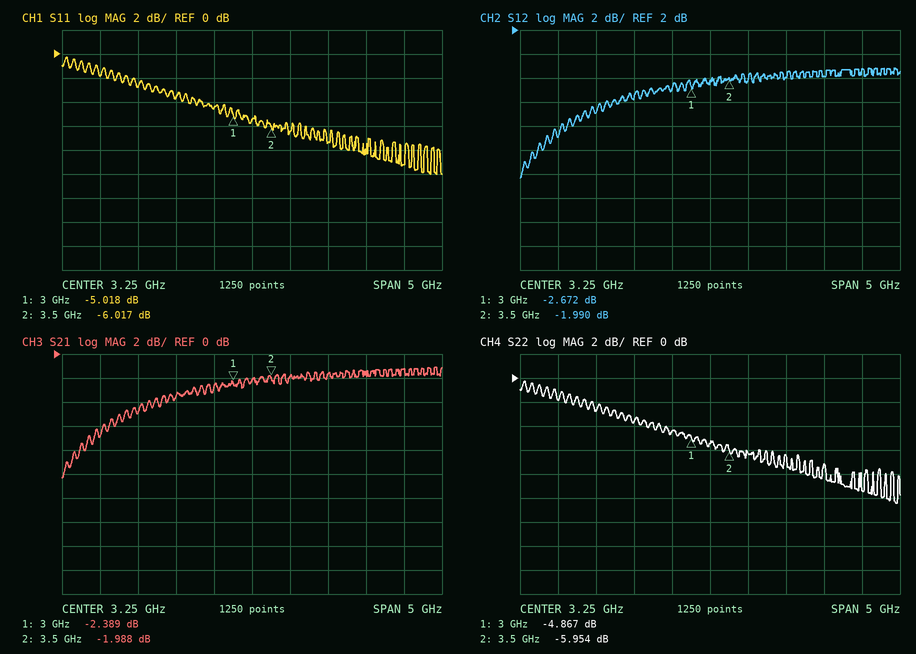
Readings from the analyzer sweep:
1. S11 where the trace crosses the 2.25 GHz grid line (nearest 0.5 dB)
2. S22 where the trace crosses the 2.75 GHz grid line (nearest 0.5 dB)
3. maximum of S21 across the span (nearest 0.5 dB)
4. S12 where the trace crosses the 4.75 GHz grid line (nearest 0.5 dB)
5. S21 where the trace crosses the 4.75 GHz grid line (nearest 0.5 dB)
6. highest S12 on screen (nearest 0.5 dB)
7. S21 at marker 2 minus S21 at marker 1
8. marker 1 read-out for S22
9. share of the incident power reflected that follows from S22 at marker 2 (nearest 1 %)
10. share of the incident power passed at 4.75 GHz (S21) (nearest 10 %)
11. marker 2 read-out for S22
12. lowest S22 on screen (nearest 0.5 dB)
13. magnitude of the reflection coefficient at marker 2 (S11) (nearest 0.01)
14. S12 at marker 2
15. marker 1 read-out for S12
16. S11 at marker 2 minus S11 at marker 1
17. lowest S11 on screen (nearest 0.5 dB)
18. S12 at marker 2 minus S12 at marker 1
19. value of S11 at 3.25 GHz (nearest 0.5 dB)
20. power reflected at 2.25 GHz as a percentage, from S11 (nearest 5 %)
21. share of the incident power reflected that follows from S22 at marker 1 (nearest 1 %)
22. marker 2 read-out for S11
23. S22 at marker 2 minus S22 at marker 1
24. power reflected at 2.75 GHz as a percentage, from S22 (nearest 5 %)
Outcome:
-3.5 dB
-4.5 dB
-1.0 dB
-2.0 dB
-1.5 dB
-1.0 dB
0.401 dB
-4.867 dB
25 %
70 %
-5.954 dB
-10.5 dB
0.50
-1.990 dB
-2.672 dB
-0.999 dB
-10.0 dB
0.682 dB
-5.5 dB
45 %
33 %
-6.017 dB
-1.087 dB
35 %
